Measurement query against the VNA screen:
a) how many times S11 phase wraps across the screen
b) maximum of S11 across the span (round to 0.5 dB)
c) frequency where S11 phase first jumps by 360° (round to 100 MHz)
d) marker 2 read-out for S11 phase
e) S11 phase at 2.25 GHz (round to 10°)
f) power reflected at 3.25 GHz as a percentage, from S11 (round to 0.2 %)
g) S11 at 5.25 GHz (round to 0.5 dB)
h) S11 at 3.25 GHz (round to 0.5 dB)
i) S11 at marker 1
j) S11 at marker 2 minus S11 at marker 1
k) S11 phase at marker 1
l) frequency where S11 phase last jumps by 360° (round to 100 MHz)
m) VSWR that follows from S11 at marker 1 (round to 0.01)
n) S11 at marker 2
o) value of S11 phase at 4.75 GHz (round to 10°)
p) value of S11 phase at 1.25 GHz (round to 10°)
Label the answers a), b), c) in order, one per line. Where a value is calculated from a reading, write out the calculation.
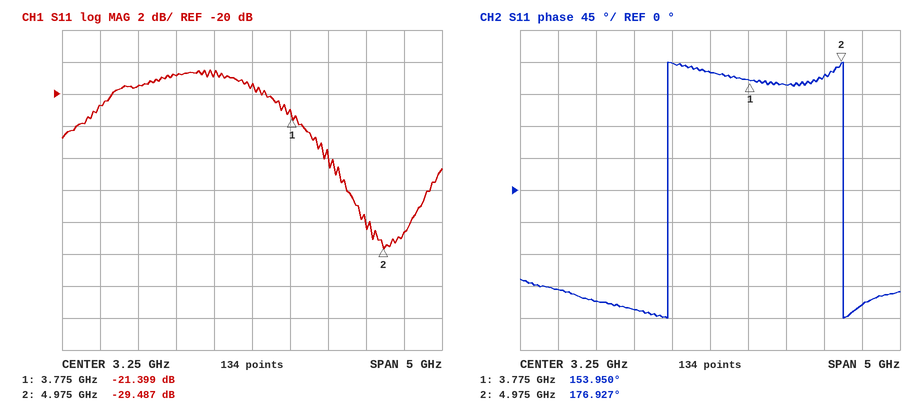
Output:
a) 2
b) -18.5 dB
c) 2.7 GHz
d) 176.927°
e) -170°
f) 10^(-19.5/10) ≈ 1.12 %, so 1.2 % to the nearest 0.2 %
g) -28.5 dB
h) -19.5 dB
i) -21.399 dB
j) -29.487 − (-21.399) = -8.088 dB
k) 153.950°
l) 5.0 GHz
m) (1 + 0.0851)/(1 − 0.0851) ≈ 1.19
n) -29.487 dB
o) 160°
p) -140°
